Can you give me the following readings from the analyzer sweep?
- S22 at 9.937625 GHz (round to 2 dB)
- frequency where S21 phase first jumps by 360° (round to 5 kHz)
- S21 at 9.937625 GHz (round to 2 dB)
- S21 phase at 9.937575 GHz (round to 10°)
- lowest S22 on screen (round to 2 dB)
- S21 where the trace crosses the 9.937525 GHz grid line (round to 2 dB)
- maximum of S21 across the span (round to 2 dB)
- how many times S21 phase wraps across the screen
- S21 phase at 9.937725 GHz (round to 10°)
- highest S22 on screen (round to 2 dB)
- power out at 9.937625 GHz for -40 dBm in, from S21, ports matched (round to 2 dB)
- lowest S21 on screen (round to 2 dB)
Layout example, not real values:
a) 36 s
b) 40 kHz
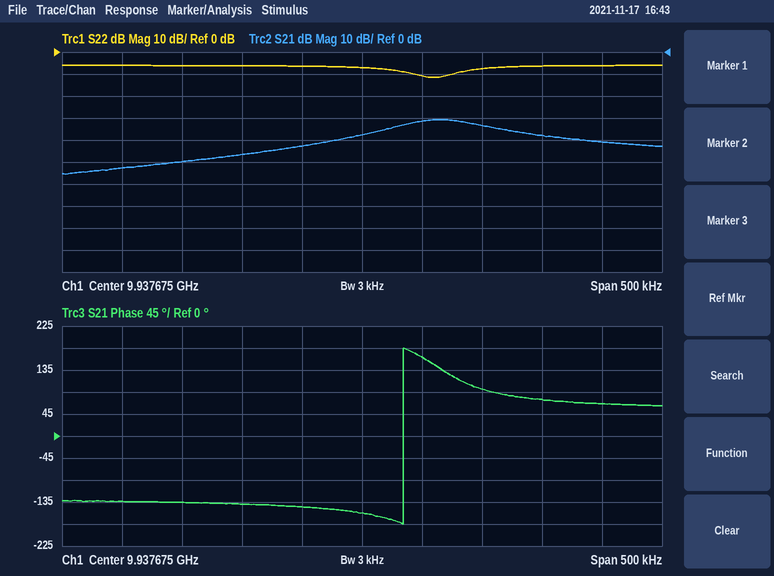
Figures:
a) -6 dB
b) 9.937710 GHz
c) -42 dB
d) -140°
e) -12 dB
f) -50 dB
g) -30 dB
h) 1
i) 160°
j) -6 dB
k) -82 dBm
l) -56 dB
